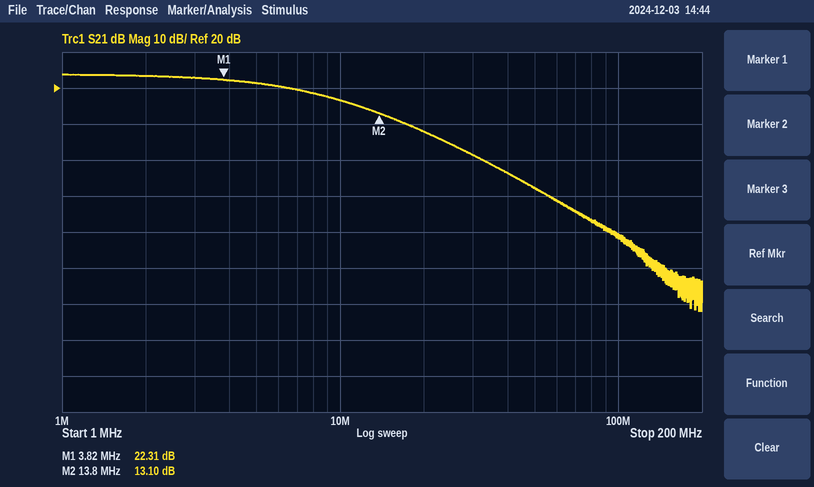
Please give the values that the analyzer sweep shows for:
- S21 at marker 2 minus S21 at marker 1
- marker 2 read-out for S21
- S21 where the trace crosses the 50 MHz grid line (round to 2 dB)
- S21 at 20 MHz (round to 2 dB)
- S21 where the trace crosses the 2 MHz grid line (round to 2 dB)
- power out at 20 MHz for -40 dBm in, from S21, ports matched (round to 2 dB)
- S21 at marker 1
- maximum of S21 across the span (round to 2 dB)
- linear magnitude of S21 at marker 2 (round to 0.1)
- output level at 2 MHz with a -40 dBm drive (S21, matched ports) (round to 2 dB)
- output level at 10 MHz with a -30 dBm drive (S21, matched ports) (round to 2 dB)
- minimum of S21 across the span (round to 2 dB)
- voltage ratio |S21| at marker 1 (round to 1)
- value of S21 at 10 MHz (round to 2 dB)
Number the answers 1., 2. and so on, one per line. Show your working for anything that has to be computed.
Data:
1. 13.1 − (22.31) = -9.21 dB
2. 13.10 dB
3. -8 dB
4. 8 dB
5. 24 dB
6. -40 dBm + (8 dB) = -32 dBm
7. 22.31 dB
8. 24 dB
9. 10^(13.1/20) ≈ 4.5
10. -40 dBm + (24 dB) = -16 dBm
11. -30 dBm + (16 dB) = -14 dBm
12. -42 dB
13. 10^(22.31/20) ≈ 13
14. 16 dB
